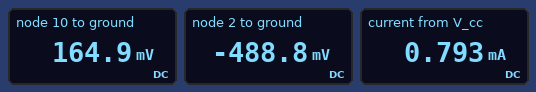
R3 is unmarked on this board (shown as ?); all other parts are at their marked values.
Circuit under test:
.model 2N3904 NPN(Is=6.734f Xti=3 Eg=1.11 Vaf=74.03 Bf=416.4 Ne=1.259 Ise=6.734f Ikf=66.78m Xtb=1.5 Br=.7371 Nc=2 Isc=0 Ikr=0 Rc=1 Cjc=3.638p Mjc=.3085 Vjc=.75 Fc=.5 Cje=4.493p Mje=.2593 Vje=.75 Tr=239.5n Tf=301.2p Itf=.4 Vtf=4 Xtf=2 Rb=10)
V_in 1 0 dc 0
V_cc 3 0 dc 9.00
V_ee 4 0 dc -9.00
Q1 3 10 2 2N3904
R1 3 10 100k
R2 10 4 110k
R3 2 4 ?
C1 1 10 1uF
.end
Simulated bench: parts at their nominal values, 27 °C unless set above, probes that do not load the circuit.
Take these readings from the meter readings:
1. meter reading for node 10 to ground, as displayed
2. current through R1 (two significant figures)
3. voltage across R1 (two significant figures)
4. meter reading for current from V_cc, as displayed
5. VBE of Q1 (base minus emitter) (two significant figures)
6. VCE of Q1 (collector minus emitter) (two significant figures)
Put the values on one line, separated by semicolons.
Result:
164.9 mV; 88 µA; 8.8 V; 0.793 mA; 650 mV; 9.5 V
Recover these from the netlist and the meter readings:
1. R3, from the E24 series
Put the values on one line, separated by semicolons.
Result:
12 kΩ
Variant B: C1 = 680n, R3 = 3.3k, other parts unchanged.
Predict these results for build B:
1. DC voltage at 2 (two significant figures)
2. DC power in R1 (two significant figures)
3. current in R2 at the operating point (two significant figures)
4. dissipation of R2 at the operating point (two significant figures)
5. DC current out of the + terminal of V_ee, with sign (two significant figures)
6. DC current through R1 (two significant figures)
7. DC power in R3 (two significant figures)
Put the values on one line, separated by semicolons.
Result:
-1.0 V; 870 µW; 79 µA; 680 µW; -2.5 mA; 93 µA; 19 mW
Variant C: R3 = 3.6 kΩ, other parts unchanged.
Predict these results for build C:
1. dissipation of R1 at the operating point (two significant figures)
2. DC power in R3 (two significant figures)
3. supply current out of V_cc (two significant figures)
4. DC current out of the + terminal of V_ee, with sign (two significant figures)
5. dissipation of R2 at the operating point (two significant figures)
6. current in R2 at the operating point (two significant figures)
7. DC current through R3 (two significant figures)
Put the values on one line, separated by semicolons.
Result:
860 µW; 18 mW; 2.3 mA; -2.3 mA; 690 µW; 79 µA; 2.2 mA
